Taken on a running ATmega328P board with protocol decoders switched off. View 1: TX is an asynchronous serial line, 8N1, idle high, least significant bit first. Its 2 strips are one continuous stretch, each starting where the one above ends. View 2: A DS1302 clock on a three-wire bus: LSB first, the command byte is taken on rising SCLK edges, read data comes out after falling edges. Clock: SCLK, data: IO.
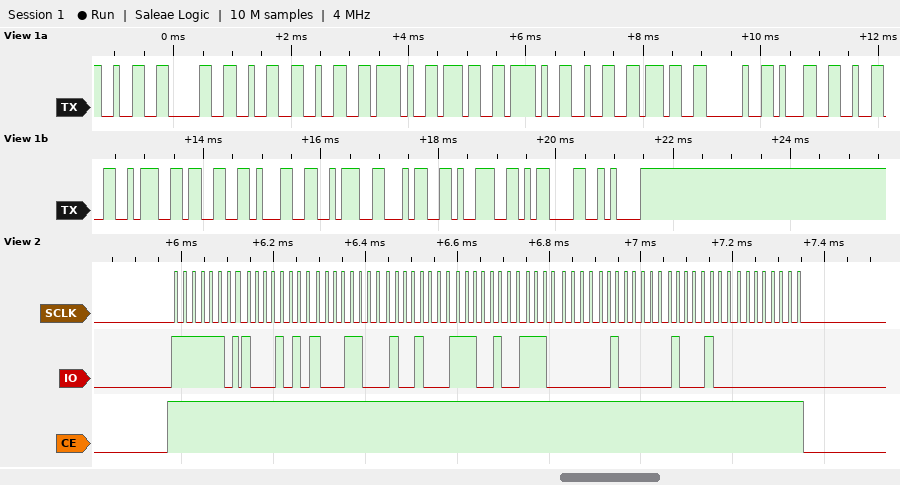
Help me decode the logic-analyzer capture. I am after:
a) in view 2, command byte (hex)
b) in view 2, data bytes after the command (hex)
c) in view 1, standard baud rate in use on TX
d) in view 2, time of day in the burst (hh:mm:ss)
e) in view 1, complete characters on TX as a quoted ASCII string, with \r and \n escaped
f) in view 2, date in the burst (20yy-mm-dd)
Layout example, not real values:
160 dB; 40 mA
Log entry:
0xBF; 51 31 12 27 07 04 22 00; 9600 baud; 12:31:51; "2022/7/27 12:31:49\r\n"; 2022-07-27
